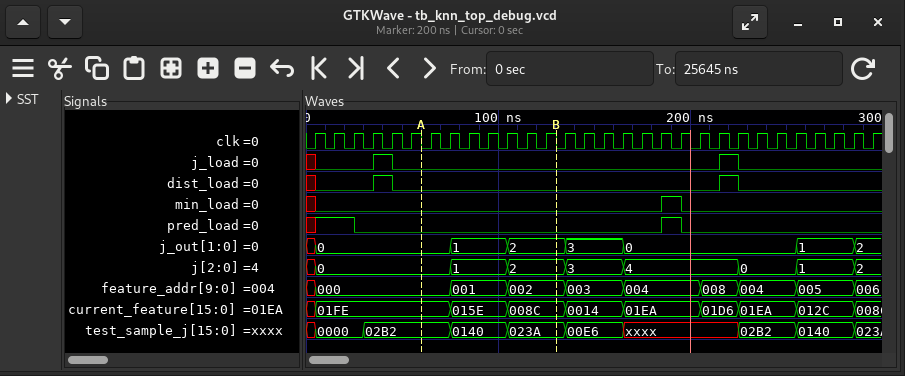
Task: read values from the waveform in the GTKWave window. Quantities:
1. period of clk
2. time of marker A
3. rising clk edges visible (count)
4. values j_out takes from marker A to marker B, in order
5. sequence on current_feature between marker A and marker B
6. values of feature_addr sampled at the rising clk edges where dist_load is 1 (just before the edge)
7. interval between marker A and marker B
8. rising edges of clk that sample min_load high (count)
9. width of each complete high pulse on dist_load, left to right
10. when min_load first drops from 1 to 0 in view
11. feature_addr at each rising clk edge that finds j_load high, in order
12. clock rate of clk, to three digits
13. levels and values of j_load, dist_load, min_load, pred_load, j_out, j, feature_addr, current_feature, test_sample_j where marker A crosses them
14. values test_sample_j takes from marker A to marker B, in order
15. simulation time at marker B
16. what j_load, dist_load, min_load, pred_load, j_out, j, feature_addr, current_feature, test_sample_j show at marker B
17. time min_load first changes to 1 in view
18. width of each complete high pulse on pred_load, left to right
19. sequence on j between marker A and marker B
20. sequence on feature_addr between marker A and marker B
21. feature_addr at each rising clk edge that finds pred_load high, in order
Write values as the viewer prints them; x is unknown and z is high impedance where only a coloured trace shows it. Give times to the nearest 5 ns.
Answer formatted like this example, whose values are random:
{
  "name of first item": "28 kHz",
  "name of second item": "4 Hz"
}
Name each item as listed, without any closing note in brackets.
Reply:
{
  "period of clk": "10 ns",
  "time of marker A": "60 ns",
  "rising clk edges visible": "30",
  "values j_out takes from marker A to marker B, in order": "0, 1, 2",
  "sequence on current_feature between marker A and marker B": "01FE, 015E, 008C",
  "values of feature_addr sampled at the rising clk edges where dist_load is 1": "000, 008",
  "interval between marker A and marker B": "70 ns",
  "rising edges of clk that sample min_load high": "1",
  "width of each complete high pulse on dist_load, left to right": "10 ns, 10 ns",
  "when min_load first drops from 1 to 0 in view": "195 ns",
  "feature_addr at each rising clk edge that finds j_load high, in order": "000, 008",
  "clock rate of clk, to three digits": "100 MHz",
  "levels and values of j_load, dist_load, min_load, pred_load, j_out, j, feature_addr, current_feature, test_sample_j where marker A crosses them": "j_load=0, dist_load=0, min_load=0, pred_load=0, j_out=0, j=0, feature_addr=000, current_feature=01FE, test_sample_j=02B2",
  "values test_sample_j takes from marker A to marker B, in order": "02B2, 0140, 023A",
  "simulation time at marker B": "130 ns",
  "what j_load, dist_load, min_load, pred_load, j_out, j, feature_addr, current_feature, test_sample_j show at marker B": "j_load=0, dist_load=0, min_load=0, pred_load=0, j_out=2, j=2, feature_addr=002, current_feature=008C, test_sample_j=023A",
  "time min_load first changes to 1 in view": "185 ns",
  "width of each complete high pulse on pred_load, left to right": "10 ns",
  "sequence on j between marker A and marker B": "0, 1, 2",
  "sequence on feature_addr between marker A and marker B": "000, 001, 002",
  "feature_addr at each rising clk edge that finds pred_load high, in order": "000, 000, 004"
}
